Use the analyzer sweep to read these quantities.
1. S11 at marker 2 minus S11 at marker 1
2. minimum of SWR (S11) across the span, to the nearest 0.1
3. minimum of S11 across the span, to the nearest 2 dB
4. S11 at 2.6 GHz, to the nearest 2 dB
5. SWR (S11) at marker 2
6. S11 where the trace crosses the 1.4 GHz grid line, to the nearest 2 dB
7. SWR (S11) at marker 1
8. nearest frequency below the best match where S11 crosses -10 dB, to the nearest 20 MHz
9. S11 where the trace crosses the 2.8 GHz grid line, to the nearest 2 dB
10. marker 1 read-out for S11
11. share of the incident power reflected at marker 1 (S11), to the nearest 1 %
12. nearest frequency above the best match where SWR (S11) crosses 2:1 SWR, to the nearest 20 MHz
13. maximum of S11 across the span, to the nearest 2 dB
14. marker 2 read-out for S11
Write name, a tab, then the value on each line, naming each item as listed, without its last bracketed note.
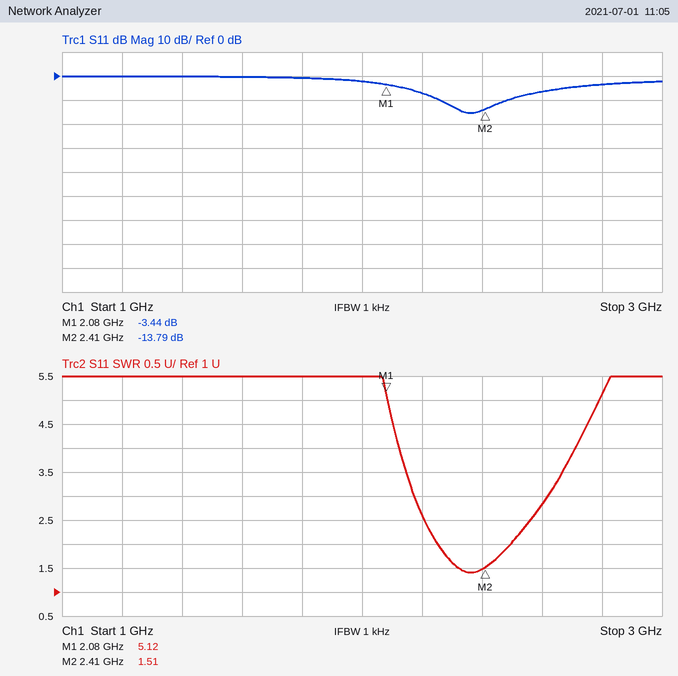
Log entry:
S11 at marker 2 minus S11 at marker 1	-10.35 dB
minimum of SWR (S11) across the span, to the nearest 0.1	1.4
minimum of S11 across the span, to the nearest 2 dB	-16 dB
S11 at 2.6 GHz, to the nearest 2 dB	-6 dB
SWR (S11) at marker 2	1.51
S11 where the trace crosses the 1.4 GHz grid line, to the nearest 2 dB	0 dB
SWR (S11) at marker 1	5.12
nearest frequency below the best match where S11 crosses -10 dB, to the nearest 20 MHz	2.26 GHz
S11 where the trace crosses the 2.8 GHz grid line, to the nearest 2 dB	-4 dB
marker 1 read-out for S11	-3.44 dB
share of the incident power reflected at marker 1 (S11), to the nearest 1 %	45 %
nearest frequency above the best match where SWR (S11) crosses 2:1 SWR, to the nearest 20 MHz	2.50 GHz
maximum of S11 across the span, to the nearest 2 dB	0 dB
marker 2 read-out for S11	-13.79 dB
